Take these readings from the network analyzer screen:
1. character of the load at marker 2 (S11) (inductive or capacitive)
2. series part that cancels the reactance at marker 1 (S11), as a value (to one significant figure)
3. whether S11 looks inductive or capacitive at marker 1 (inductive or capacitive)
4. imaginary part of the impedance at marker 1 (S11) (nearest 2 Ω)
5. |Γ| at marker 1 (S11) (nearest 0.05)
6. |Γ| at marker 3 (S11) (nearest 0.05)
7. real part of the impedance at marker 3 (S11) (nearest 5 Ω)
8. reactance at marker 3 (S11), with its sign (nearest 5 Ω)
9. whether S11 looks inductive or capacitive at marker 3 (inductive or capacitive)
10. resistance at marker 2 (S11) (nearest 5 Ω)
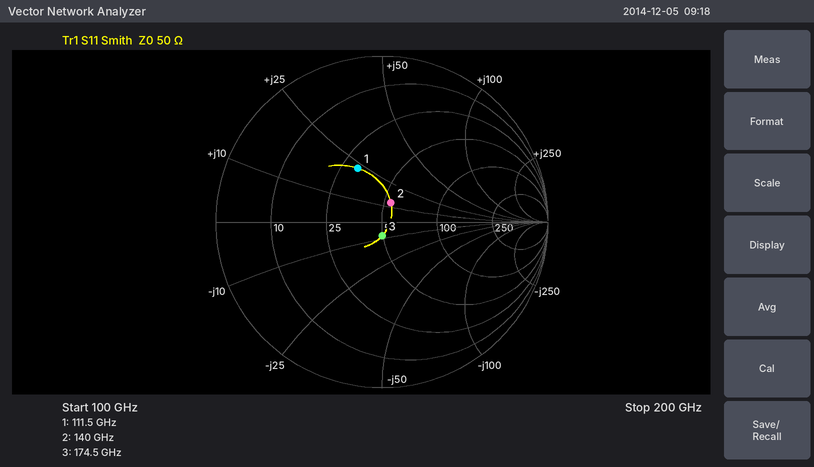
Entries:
inductive
60 fF
inductive
+22 Ω
0.35
0.10
50 Ω
-10 Ω
capacitive
55 Ω
